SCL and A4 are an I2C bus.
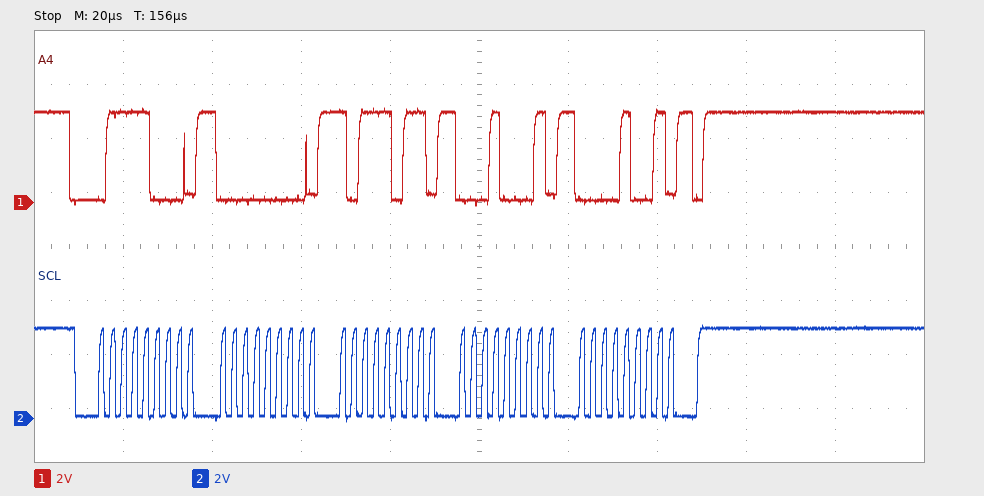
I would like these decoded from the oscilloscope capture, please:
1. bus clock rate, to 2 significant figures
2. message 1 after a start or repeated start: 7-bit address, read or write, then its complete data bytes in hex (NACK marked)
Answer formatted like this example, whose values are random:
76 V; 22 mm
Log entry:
400 kHz; 0x3C write: 00 BB 11 09
